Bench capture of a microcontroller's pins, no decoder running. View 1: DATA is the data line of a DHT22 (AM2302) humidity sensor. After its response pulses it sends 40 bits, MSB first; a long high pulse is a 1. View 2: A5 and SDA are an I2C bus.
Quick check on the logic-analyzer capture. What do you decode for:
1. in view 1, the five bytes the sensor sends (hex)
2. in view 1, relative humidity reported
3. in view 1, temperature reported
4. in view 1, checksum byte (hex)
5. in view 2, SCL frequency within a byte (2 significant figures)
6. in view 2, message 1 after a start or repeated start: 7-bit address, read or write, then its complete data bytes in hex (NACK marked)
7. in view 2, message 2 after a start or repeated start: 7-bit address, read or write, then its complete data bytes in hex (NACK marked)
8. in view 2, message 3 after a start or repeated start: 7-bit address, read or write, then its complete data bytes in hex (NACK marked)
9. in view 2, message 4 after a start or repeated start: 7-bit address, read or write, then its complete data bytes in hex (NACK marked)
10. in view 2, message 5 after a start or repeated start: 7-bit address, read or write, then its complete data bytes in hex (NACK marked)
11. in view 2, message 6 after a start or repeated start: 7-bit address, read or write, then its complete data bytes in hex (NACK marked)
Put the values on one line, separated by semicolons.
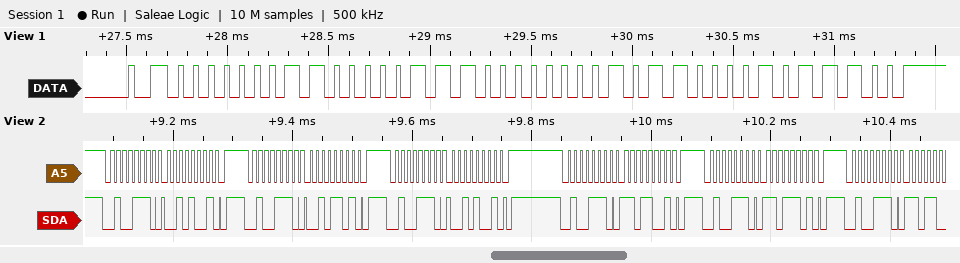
01 83 80 58 5C; 38.7 %; -8.8 °C; 0x5C; 100 kHz; 0x27 write: 29; 0x27 write: 2D; 0x27 write: 29; 0x27 write: D9; 0x27 write: DD; 0x27 write
